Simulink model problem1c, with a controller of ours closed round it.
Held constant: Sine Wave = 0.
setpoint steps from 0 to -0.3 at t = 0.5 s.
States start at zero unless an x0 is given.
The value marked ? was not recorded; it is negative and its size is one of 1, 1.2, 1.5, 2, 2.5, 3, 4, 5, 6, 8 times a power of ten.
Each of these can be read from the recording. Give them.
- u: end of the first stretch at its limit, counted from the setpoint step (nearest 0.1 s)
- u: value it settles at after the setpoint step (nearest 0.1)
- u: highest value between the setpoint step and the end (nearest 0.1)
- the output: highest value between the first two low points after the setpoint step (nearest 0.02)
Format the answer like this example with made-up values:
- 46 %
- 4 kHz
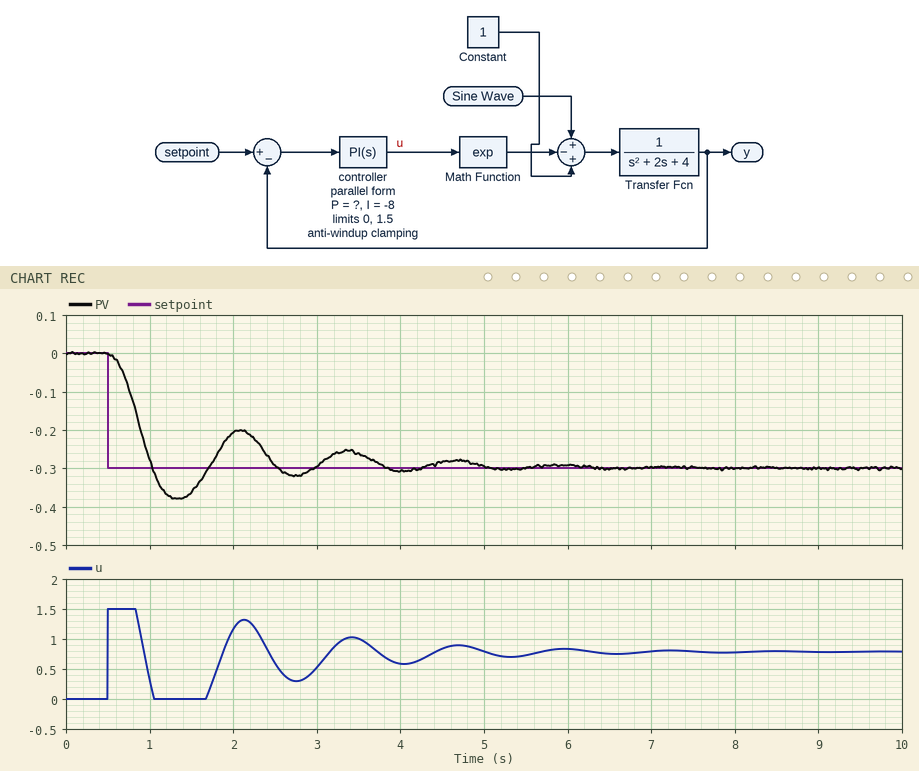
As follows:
- 0.3 s
- 0.8
- 1.5
- -0.20
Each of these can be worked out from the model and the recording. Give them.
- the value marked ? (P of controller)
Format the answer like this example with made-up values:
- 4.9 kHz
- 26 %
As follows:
- -10
